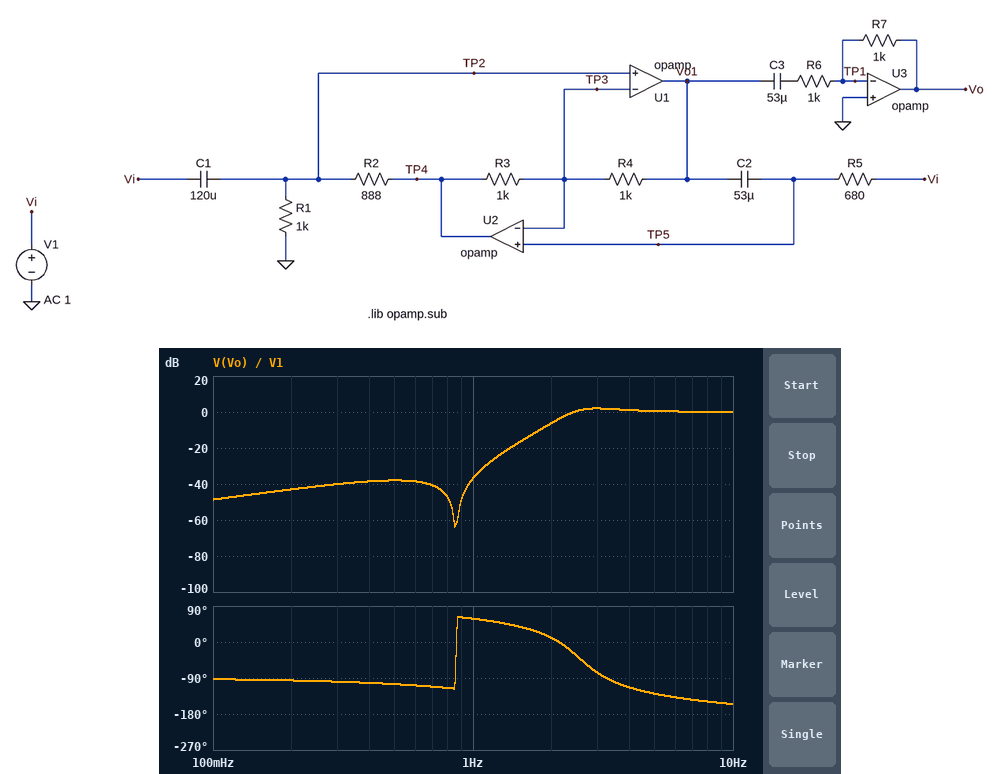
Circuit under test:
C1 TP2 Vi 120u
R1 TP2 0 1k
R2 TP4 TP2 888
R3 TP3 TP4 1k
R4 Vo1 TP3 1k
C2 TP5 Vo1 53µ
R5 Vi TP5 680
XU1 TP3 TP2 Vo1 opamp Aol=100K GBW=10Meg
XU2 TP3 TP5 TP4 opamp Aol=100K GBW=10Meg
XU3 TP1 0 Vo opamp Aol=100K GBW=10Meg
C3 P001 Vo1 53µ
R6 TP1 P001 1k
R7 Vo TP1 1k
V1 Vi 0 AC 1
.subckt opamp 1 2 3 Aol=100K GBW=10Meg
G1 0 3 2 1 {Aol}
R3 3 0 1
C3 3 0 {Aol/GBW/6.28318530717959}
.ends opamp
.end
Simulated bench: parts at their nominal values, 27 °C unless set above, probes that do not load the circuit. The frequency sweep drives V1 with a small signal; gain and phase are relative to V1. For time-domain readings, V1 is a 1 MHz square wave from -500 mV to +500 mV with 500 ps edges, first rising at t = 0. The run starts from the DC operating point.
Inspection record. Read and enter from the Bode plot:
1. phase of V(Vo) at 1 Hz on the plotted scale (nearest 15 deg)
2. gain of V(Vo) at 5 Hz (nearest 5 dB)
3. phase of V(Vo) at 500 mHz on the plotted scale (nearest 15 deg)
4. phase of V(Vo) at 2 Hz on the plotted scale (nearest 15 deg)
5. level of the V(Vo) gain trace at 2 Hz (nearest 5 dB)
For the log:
60 deg
0 dB
-105 deg
15 deg
-5 dB
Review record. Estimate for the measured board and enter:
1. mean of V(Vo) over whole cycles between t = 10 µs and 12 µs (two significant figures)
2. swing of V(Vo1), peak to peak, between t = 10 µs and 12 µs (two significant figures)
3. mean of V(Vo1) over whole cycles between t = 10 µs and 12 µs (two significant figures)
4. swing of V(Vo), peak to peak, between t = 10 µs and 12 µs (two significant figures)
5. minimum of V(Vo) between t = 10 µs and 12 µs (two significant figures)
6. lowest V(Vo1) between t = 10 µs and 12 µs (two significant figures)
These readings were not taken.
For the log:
-500 mV
1.4 V
440 mV
1.1 V
-1.0 V
-260 mV
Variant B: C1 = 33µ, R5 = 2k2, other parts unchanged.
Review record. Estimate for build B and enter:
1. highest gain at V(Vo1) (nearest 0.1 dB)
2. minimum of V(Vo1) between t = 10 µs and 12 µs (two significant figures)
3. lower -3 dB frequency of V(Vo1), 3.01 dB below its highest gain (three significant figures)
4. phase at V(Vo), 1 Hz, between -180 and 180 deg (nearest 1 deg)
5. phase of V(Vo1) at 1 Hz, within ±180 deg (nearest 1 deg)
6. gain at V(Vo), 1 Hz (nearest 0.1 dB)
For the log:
0 dB
-260 mV
3.91 Hz
35 deg
143 deg
-43.5 dB
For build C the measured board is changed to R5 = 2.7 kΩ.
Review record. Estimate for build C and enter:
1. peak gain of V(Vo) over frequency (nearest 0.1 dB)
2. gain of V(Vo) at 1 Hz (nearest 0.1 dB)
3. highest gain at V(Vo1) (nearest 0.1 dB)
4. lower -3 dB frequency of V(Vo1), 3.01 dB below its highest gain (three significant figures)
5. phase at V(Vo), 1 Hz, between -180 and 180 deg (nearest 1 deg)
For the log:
0 dB
-15.2 dB
0.7 dB
1.18 Hz
8 deg
